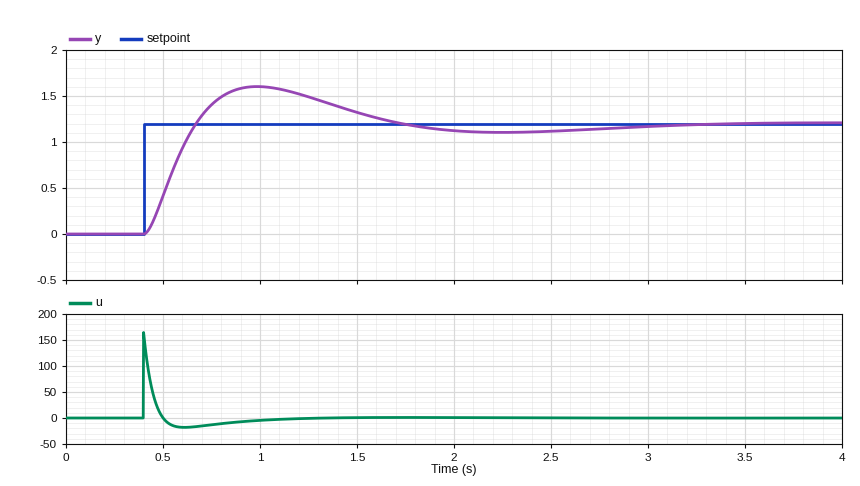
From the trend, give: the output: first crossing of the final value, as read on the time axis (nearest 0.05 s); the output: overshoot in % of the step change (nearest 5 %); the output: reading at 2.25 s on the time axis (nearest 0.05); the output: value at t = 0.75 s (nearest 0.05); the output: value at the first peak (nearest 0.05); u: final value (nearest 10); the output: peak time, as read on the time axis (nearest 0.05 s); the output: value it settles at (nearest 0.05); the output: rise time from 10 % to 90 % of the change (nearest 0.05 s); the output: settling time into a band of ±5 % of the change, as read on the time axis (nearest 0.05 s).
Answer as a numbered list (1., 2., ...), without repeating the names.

1. 0.65 s
2. 35 %
3. 1.10
4. 1.40
5. 1.60
6. 0
7. 1.00 s
8. 1.20
9. 0.20 s
10. 2.75 s
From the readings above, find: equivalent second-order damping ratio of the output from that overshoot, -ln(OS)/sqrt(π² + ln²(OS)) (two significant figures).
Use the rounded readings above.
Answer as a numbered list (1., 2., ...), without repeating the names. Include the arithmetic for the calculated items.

1. ln(0.35) = -1.050; 1.050 / sqrt(9.870 + 1.102) = 0.32
